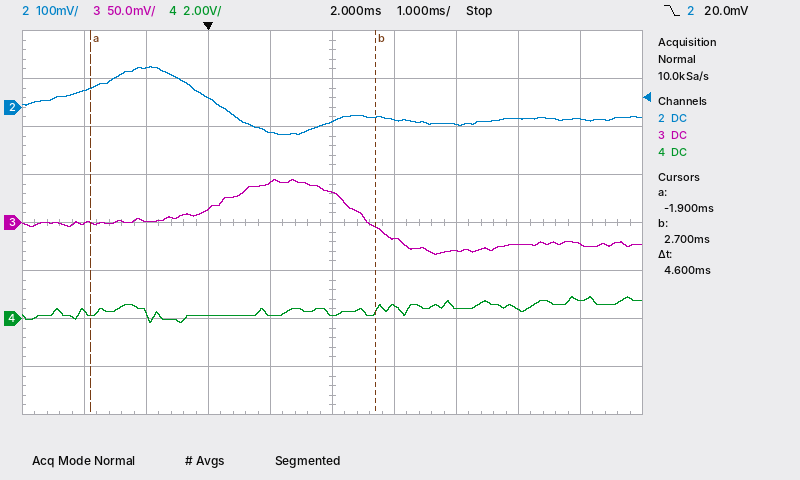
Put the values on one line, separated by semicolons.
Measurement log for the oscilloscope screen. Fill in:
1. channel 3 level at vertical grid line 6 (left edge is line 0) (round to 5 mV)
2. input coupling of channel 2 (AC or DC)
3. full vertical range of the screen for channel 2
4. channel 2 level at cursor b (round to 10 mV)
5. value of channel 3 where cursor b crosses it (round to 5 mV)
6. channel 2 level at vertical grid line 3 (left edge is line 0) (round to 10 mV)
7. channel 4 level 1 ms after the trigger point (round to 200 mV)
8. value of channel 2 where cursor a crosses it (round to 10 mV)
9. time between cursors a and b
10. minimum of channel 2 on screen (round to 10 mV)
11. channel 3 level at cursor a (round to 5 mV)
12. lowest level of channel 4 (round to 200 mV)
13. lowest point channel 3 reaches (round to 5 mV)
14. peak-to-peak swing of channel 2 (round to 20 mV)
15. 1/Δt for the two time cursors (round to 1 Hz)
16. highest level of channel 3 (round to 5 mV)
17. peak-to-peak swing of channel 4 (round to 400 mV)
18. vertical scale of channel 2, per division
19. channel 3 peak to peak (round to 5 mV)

-15 mV; DC; 800 mV; -20 mV; -5 mV; 20 mV; 200 mV; 40 mV; 4.6 ms; -60 mV; 0 mV; -200 mV; -35 mV; 140 mV; 217 Hz; 45 mV; 1.2 V; 100 mV; 80 mV
